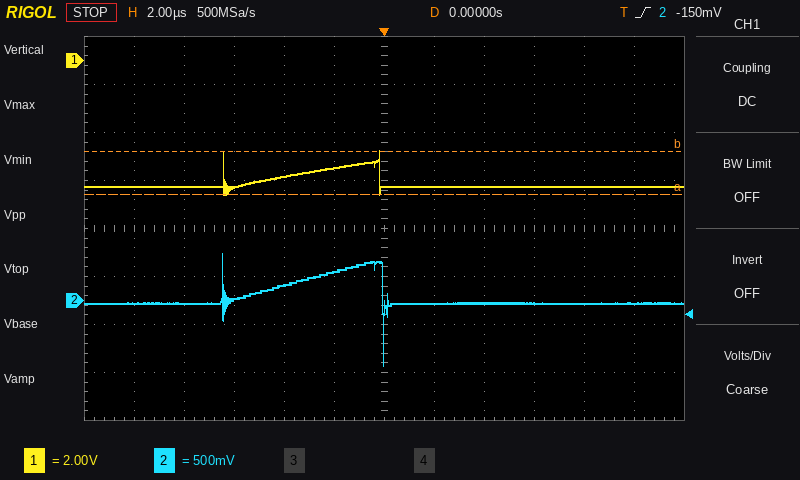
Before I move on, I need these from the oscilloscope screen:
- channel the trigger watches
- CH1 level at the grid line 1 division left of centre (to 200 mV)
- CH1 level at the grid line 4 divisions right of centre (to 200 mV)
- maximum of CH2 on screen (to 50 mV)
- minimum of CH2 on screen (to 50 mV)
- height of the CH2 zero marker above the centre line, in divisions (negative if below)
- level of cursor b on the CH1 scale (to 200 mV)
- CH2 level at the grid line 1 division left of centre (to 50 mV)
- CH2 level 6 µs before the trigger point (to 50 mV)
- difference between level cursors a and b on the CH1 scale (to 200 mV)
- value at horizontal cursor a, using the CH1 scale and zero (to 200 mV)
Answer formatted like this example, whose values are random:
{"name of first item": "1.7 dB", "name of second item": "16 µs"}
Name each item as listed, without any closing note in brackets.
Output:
{"channel the trigger watches": "CH2", "CH1 level at the grid line 1 division left of centre": "-4.4 V", "CH1 level at the grid line 4 divisions right of centre": "-5.2 V", "maximum of CH2 on screen": "500 mV", "minimum of CH2 on screen": "-700 mV", "height of the CH2 zero marker above the centre line, in divisions": "-1.5 div", "level of cursor b on the CH1 scale": "-3.8 V", "CH2 level at the grid line 1 division left of centre": "300 mV", "CH2 level 6 µs before the trigger point": "0 mV", "difference between level cursors a and b on the CH1 scale": "1.8 V", "value at horizontal cursor a, using the CH1 scale and zero": "-5.6 V"}
